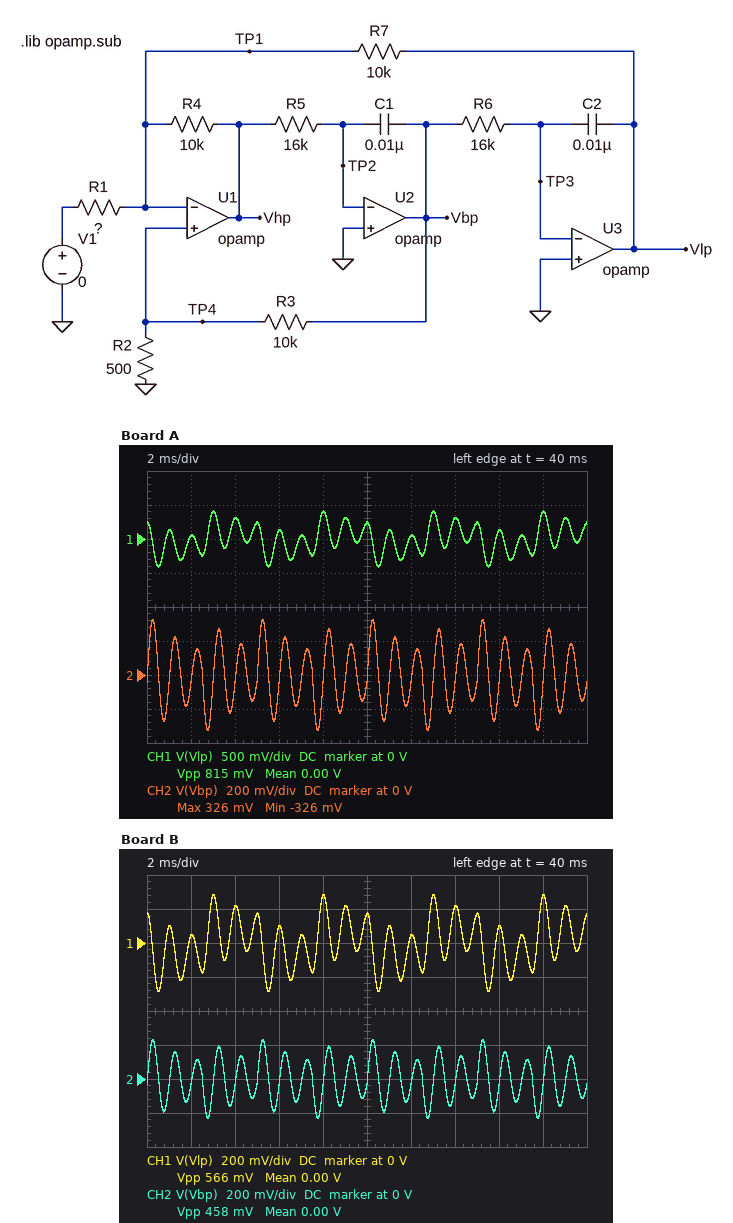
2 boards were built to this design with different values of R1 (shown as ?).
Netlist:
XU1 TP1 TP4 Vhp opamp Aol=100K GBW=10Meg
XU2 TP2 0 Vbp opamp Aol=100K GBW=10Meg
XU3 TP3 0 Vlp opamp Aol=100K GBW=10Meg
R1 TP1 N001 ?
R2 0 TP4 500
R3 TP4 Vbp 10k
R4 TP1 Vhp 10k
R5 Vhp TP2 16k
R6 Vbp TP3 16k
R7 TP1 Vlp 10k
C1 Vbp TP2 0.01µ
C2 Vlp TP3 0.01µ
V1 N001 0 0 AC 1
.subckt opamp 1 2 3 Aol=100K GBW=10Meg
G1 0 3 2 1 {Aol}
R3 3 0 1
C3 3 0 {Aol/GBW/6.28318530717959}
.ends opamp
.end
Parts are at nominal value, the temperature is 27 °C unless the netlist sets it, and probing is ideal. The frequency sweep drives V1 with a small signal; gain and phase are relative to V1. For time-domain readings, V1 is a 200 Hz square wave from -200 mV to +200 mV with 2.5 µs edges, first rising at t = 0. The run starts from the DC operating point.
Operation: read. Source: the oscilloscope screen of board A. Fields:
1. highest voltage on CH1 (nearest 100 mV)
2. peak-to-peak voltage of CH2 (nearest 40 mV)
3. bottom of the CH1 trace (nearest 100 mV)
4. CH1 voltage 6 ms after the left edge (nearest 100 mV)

400 mV
640 mV
-400 mV
100 mV
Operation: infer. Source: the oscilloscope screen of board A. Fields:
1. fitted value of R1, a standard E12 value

18 kΩ
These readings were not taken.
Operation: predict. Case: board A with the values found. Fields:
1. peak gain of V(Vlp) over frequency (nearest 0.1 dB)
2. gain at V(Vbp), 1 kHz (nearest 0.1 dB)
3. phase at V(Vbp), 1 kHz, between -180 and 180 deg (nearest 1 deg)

13.2 dB
13.2 dB
-5 deg
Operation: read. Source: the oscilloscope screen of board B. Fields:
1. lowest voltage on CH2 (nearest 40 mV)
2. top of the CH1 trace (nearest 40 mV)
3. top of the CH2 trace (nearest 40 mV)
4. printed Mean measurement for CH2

-240 mV
280 mV
240 mV
0.00 V
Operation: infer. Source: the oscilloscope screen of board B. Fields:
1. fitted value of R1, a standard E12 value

27 kΩ
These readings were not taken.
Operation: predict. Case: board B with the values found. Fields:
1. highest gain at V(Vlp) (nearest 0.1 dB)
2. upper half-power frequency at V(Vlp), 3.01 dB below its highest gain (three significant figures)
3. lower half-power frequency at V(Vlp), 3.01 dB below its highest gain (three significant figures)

10.4 dB
1.05 kHz
934 Hz
